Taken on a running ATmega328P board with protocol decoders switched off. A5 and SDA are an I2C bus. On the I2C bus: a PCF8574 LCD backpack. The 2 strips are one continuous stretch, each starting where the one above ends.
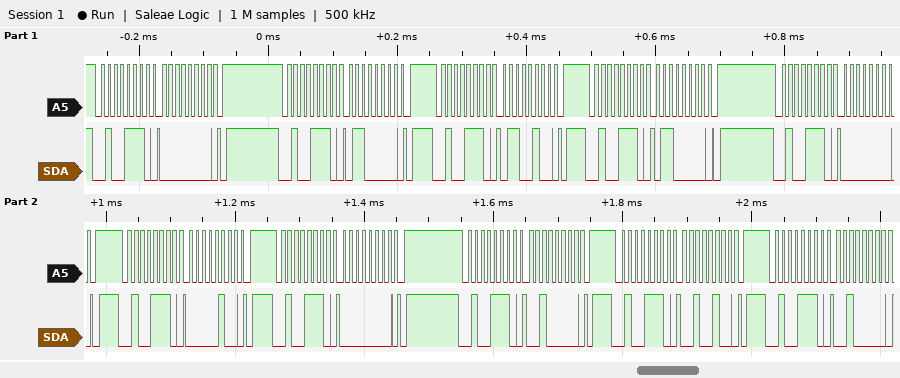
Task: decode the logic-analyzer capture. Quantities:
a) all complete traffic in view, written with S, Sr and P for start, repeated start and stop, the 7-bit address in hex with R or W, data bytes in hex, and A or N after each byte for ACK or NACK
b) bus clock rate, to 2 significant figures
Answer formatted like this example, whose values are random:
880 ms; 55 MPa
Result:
S 27W A 00 A P S 27W A 60 A P S 27W A 64 A P S 27W A 60 A P S 27W A 00 A P S 27W A 04 A P S 27W A 00 A P S 27W A 20 A P S 27W A 24 A P S 27W A 20 A; 100 kHz
